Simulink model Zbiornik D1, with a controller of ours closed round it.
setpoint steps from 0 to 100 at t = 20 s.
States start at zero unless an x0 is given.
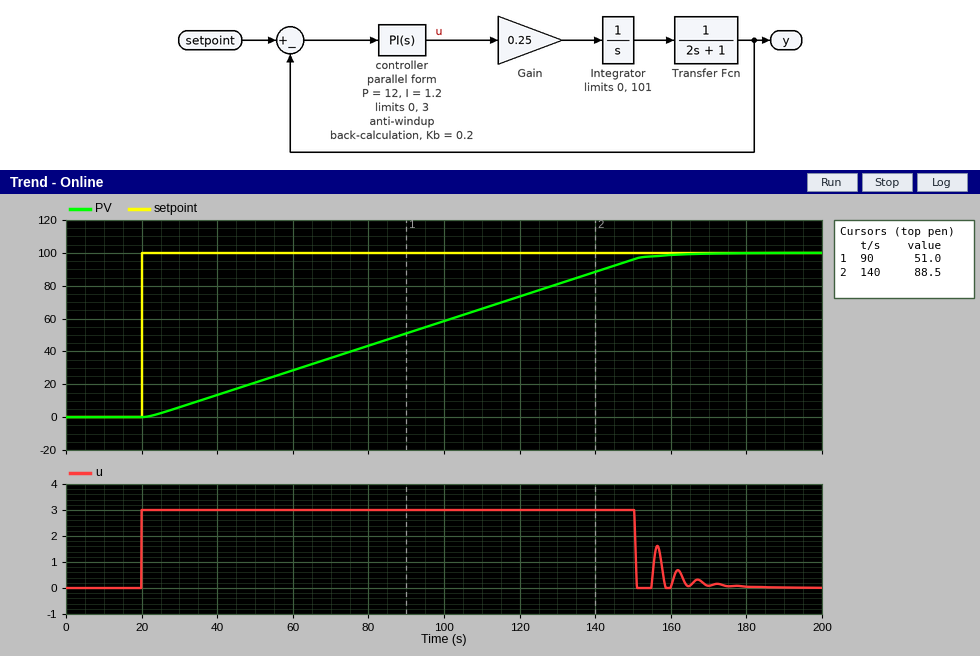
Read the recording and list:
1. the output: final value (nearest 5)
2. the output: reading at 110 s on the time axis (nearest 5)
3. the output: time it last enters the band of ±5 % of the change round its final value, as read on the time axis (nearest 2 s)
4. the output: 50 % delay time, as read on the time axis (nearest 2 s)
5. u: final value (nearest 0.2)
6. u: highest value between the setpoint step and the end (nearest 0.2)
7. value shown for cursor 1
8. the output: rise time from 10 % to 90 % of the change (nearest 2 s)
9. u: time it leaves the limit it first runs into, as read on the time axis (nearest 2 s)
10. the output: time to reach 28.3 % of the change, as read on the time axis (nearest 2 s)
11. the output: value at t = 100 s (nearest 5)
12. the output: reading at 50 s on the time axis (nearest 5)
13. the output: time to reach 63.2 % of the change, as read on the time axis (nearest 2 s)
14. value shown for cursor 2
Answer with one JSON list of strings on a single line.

["100", "65", "148 s", "88 s", "0.0", "3.0", "51.0", "106 s", "150 s", "60 s", "60", "20", "106 s", "88.5"]
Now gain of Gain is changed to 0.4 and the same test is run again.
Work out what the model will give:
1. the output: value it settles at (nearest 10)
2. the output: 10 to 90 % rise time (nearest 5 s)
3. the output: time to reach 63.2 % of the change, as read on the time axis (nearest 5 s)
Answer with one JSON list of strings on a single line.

["100", "65 s", "75 s"]
